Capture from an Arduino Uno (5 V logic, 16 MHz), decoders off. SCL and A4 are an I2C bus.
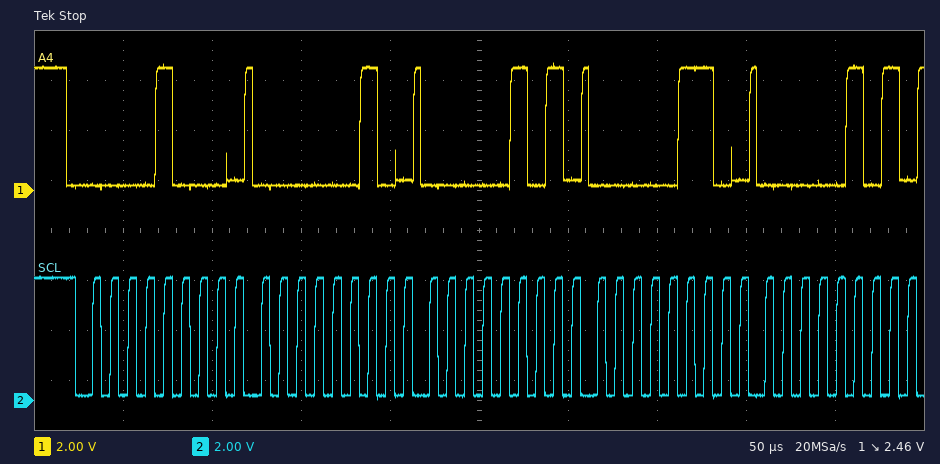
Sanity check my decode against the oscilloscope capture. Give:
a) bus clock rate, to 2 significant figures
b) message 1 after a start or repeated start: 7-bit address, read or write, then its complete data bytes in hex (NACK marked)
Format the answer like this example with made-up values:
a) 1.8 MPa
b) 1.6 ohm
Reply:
a) 100 kHz
b) 0x04 write: 02 05 06 05
